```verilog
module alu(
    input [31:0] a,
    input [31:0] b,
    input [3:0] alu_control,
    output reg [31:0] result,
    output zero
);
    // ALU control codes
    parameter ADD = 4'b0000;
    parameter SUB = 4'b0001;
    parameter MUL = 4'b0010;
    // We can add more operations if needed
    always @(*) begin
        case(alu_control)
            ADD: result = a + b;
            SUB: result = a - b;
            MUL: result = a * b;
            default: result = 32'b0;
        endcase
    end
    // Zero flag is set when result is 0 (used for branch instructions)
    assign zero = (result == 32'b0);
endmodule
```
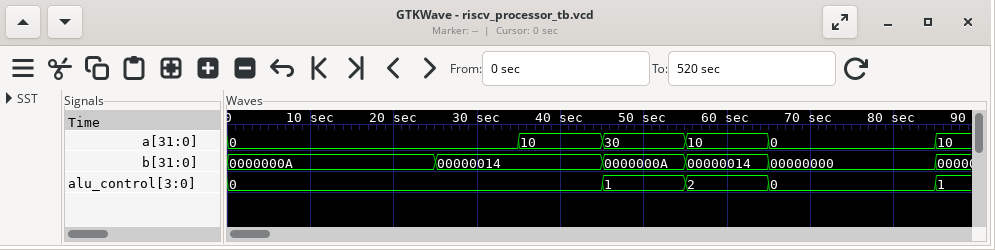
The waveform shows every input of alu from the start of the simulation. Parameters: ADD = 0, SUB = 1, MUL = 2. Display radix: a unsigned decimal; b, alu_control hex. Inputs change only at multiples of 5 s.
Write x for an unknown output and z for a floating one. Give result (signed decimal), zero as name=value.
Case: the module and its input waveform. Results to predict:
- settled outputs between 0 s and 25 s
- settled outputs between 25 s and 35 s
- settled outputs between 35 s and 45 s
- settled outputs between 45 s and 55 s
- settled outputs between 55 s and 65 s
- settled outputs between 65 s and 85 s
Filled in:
result=10, zero=0
result=20, zero=0
result=30, zero=0
result=20, zero=0
result=200, zero=0
result=0, zero=1
